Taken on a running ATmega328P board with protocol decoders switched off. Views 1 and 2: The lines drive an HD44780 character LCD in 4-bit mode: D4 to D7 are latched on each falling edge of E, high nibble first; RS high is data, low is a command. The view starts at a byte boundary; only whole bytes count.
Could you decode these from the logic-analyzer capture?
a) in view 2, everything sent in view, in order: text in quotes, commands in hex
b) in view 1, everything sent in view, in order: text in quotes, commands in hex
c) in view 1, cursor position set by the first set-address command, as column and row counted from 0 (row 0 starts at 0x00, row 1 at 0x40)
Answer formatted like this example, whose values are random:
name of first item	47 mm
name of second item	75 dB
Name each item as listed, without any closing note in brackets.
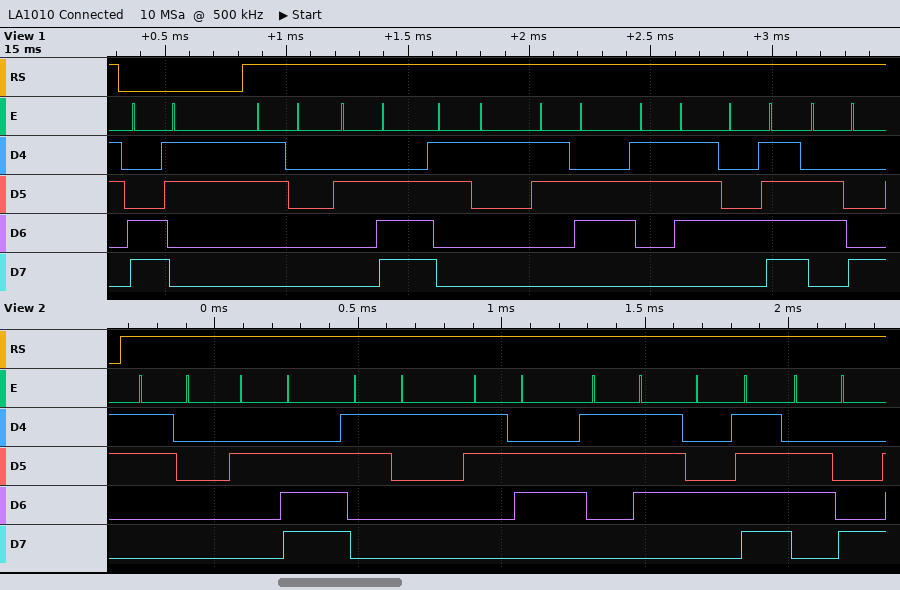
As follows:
in view 2, everything sent in view, in order: text in quotes, commands in hex	"0.167Oh"
in view 1, everything sent in view, in order: text in quotes, commands in hex	0xC3 "0.167Oh"
in view 1, cursor position set by the first set-address command, as column and row counted from 0	column 3, row 1
